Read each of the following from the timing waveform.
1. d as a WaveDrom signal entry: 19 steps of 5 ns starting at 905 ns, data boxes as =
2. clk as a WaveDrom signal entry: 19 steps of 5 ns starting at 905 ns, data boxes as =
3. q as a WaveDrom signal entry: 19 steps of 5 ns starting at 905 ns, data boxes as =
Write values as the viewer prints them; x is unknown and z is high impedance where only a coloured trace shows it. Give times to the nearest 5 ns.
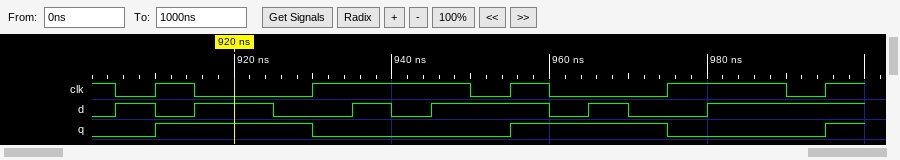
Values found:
{name: 'd', wave: '101.0.101..010.1...'}
{name: 'clk', wave: '010..1...010..1..01'}
{name: 'q', wave: '01...0....1...0...1'}
